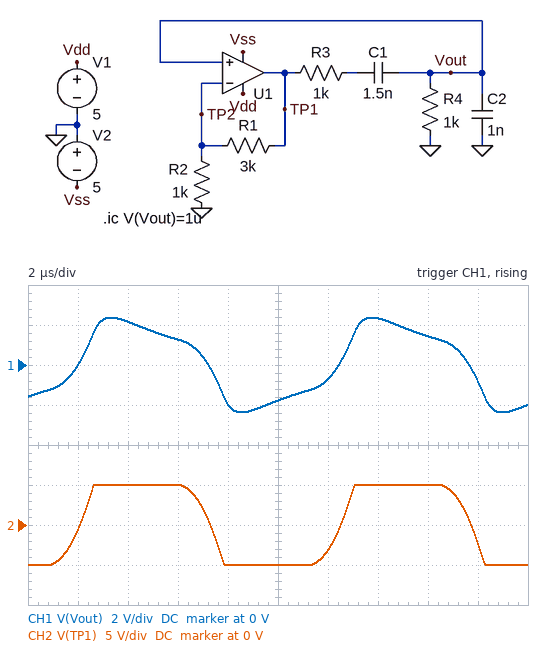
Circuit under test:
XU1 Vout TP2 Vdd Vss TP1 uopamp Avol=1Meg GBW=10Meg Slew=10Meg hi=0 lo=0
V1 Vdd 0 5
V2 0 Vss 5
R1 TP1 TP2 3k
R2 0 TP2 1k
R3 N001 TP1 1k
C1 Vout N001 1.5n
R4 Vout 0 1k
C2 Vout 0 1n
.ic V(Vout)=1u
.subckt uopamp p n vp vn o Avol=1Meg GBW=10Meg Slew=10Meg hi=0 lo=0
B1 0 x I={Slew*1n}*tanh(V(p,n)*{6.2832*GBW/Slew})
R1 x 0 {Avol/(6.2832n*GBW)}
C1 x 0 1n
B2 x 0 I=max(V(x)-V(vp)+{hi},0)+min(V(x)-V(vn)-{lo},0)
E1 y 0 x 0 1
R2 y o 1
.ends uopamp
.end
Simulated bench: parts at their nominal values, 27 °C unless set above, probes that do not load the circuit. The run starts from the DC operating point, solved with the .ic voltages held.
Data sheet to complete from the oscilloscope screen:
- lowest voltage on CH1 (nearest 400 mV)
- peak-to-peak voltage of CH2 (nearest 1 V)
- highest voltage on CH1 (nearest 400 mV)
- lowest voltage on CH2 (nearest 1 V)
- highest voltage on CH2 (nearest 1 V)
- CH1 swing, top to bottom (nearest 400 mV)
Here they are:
-2.4 V
10 V
2.4 V
-5 V
5 V
4.8 V
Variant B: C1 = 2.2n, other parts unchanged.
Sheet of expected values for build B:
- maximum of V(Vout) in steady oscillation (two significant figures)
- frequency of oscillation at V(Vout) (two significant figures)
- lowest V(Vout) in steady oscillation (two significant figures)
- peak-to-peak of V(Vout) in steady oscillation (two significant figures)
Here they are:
2.7 V
72 kHz
-2.7 V
5.3 V
